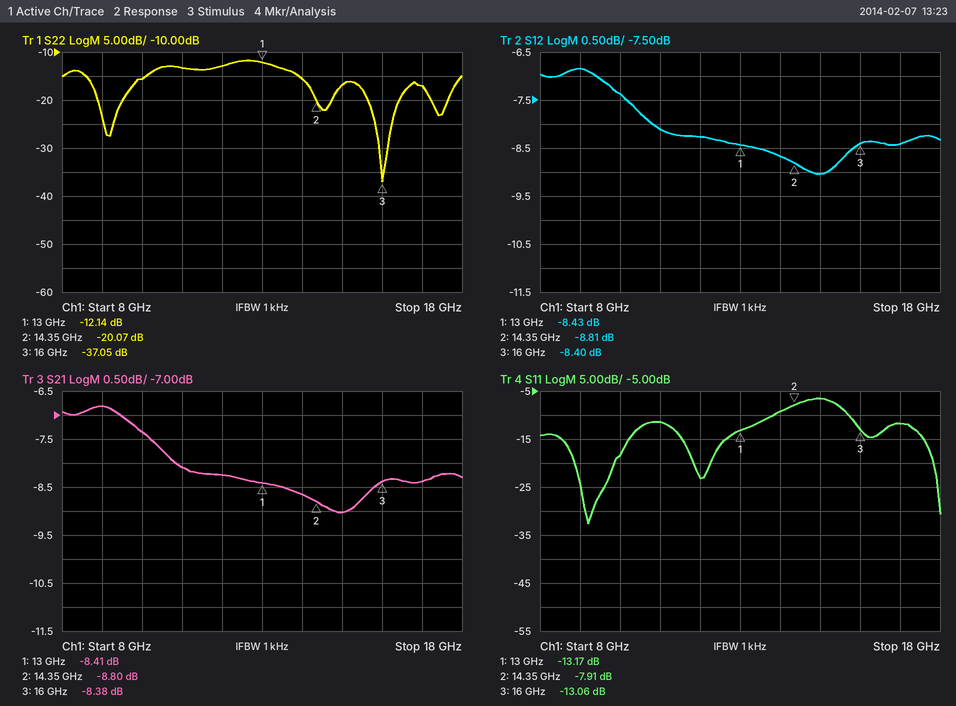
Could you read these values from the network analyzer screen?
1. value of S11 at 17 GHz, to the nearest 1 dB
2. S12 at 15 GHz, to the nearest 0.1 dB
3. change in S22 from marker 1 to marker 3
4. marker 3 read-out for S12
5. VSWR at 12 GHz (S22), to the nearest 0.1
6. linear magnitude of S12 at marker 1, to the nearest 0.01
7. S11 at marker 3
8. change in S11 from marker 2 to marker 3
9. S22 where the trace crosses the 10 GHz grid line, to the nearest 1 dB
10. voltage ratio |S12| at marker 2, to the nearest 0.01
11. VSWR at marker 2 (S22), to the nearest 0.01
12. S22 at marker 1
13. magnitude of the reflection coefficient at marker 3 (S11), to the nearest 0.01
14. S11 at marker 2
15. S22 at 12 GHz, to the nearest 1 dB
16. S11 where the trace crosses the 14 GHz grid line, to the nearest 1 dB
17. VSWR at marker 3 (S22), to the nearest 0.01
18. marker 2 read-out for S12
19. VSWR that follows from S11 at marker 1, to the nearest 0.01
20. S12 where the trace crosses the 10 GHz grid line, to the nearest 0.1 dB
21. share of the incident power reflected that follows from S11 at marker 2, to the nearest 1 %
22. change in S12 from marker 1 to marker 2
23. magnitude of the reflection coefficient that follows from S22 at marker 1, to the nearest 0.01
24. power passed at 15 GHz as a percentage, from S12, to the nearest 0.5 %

-12 dB
-9.0 dB
-24.91 dB
-8.40 dB
1.6
0.38
-13.06 dB
-5.15 dB
-16 dB
0.36
1.22
-12.14 dB
0.22
-7.91 dB
-13 dB
-9 dB
1.03
-8.81 dB
1.56
-7.4 dB
16 %
-0.38 dB
0.25
12.5 %
